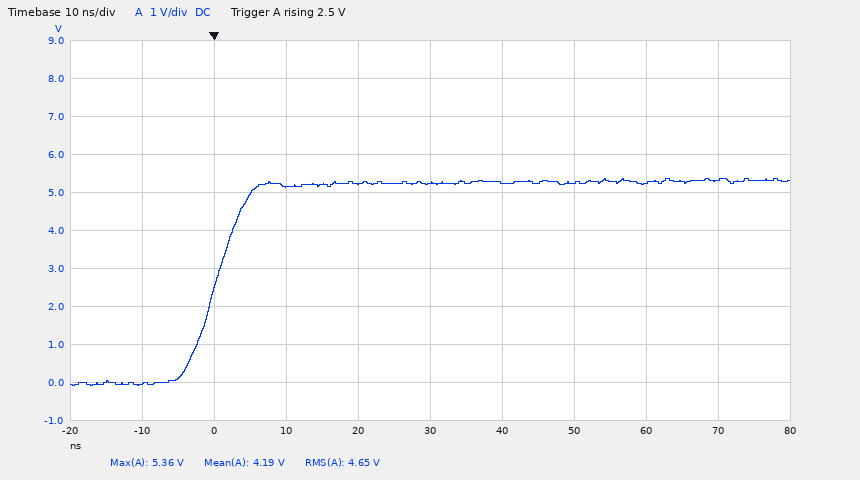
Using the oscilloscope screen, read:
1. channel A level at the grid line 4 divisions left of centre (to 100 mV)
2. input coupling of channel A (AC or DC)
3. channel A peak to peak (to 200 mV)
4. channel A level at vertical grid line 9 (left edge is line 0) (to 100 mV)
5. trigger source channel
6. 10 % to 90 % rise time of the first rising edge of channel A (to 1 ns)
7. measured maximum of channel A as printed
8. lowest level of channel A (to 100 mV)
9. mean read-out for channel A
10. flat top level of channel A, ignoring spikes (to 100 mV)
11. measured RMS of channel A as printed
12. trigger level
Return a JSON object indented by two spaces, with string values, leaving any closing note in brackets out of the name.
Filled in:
{
  "channel A level at the grid line 4 divisions left of centre": "0.0 V",
  "input coupling of channel A": "DC",
  "channel A peak to peak": "5.4 V",
  "channel A level at vertical grid line 9 (left edge is line 0)": "5.3 V",
  "trigger source channel": "channel A",
  "10 % to 90 % rise time of the first rising edge of channel A": "8 ns",
  "measured maximum of channel A as printed": "5.36 V",
  "lowest level of channel A": "-100 mV",
  "mean read-out for channel A": "4.19 V",
  "flat top level of channel A, ignoring spikes": "5.3 V",
  "measured RMS of channel A as printed": "4.65 V",
  "trigger level": "2.5 V"
}
